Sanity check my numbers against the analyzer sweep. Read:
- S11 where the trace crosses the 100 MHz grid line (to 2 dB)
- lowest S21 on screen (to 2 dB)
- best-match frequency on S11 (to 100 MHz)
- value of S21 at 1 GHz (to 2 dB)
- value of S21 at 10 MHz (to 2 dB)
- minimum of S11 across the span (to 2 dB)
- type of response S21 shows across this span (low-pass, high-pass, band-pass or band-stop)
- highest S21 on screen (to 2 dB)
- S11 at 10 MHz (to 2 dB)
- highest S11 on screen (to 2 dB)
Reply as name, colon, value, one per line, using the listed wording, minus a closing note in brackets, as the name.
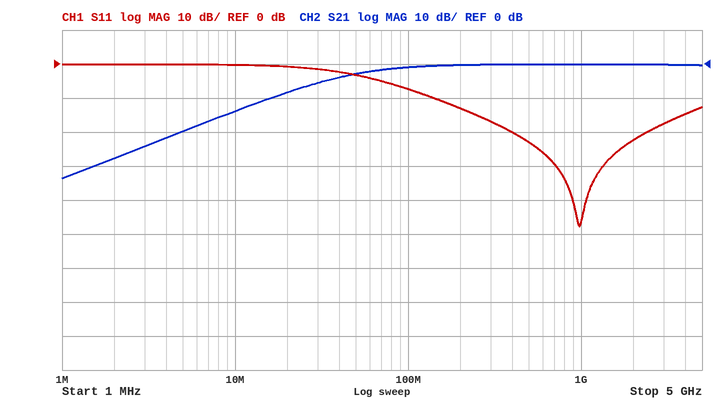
S11 where the trace crosses the 100 MHz grid line: -8 dB
lowest S21 on screen: -34 dB
best-match frequency on S11: 1.0 GHz
value of S21 at 1 GHz: 0 dB
value of S21 at 10 MHz: -14 dB
minimum of S11 across the span: -48 dB
type of response S21 shows across this span: high-pass
highest S21 on screen: 0 dB
S11 at 10 MHz: 0 dB
highest S11 on screen: 0 dB
